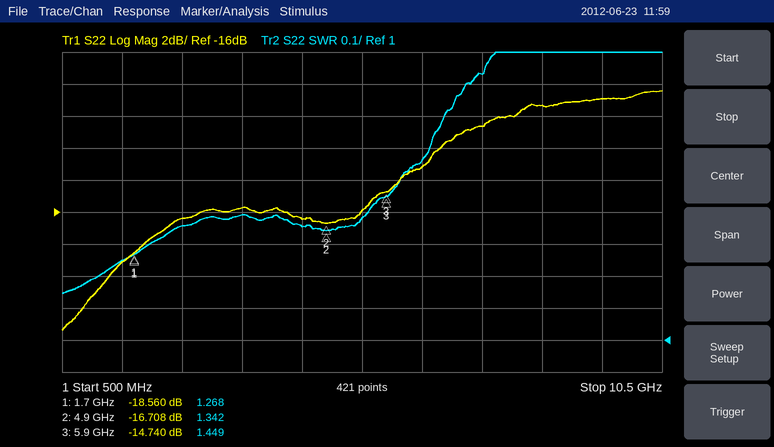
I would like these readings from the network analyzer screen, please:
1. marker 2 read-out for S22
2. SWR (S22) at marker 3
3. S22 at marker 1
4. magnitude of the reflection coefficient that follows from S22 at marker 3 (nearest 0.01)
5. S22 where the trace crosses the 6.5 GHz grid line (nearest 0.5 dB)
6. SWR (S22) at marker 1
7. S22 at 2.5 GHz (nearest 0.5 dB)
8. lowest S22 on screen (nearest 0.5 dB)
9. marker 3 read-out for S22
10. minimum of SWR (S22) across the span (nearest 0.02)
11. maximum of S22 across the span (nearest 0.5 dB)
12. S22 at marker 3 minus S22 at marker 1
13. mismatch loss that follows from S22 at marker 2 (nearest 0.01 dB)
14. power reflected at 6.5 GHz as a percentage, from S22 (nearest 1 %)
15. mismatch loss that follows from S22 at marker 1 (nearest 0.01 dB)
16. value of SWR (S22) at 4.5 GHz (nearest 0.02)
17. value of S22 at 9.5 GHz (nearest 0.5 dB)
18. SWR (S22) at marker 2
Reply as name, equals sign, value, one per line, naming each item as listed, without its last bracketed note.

marker 2 read-out for S22 = -16.708 dB
SWR (S22) at marker 3 = 1.449
S22 at marker 1 = -18.560 dB
magnitude of the reflection coefficient that follows from S22 at marker 3 = 0.18
S22 where the trace crosses the 6.5 GHz grid line = -13.0 dB
SWR (S22) at marker 1 = 1.268
S22 at 2.5 GHz = -16.5 dB
lowest S22 on screen = -23.5 dB
marker 3 read-out for S22 = -14.740 dB
minimum of SWR (S22) across the span = 1.14
maximum of S22 across the span = -8.5 dB
S22 at marker 3 minus S22 at marker 1 = 3.820 dB
mismatch loss that follows from S22 at marker 2 = 0.09 dB
power reflected at 6.5 GHz as a percentage, from S22 = 5 %
mismatch loss that follows from S22 at marker 1 = 0.06 dB
value of SWR (S22) at 4.5 GHz = 1.36
value of S22 at 9.5 GHz = -9.0 dB
SWR (S22) at marker 2 = 1.342
